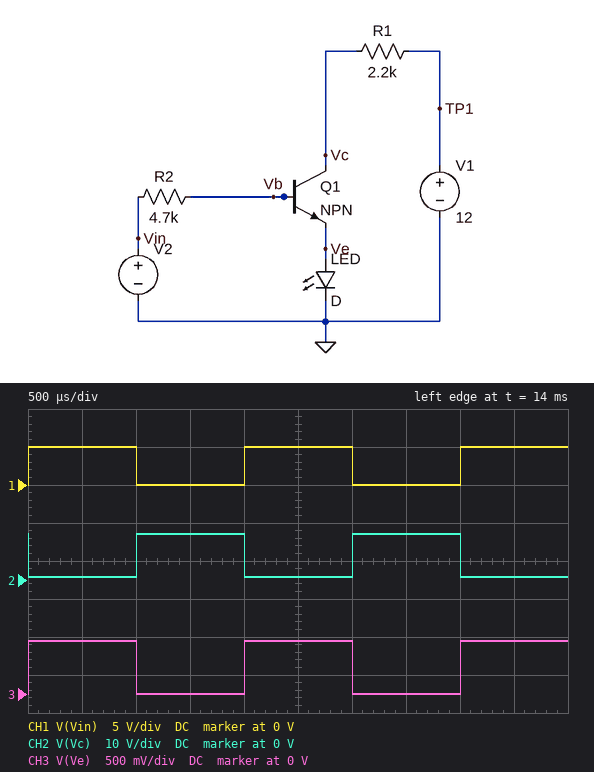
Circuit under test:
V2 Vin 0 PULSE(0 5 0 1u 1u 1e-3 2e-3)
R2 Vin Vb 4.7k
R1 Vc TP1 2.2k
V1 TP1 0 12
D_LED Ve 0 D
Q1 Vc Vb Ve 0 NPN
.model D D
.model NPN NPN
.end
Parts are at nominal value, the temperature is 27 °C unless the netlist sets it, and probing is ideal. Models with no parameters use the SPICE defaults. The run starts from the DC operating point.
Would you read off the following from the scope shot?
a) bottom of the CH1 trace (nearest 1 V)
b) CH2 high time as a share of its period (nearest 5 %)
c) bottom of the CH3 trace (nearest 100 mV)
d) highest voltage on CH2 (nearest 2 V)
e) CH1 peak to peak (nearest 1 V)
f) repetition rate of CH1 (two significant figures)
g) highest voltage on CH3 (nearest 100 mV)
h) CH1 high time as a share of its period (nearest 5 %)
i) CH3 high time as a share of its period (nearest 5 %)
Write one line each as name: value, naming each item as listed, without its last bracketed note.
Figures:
bottom of the CH1 trace: 0 V
CH2 high time as a share of its period: 50 %
bottom of the CH3 trace: 0 V
highest voltage on CH2: 12 V
CH1 peak to peak: 5 V
repetition rate of CH1: 500 Hz
highest voltage on CH3: 700 mV
CH1 high time as a share of its period: 50 %
CH3 high time as a share of its period: 50 %
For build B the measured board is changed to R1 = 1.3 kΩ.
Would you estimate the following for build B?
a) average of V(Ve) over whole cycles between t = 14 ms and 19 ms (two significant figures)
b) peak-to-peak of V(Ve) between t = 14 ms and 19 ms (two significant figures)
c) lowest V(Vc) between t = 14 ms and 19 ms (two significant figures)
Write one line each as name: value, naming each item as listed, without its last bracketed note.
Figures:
average of V(Ve) over whole cycles between t = 14 ms and 19 ms: 360 mV
peak-to-peak of V(Ve) between t = 14 ms and 19 ms: 710 mV
lowest V(Vc) between t = 14 ms and 19 ms: 780 mV
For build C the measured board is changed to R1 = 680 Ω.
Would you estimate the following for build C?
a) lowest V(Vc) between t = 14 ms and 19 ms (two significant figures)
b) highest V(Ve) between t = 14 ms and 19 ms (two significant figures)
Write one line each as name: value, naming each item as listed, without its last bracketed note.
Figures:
lowest V(Vc) between t = 14 ms and 19 ms: 820 mV
highest V(Ve) between t = 14 ms and 19 ms: 730 mV
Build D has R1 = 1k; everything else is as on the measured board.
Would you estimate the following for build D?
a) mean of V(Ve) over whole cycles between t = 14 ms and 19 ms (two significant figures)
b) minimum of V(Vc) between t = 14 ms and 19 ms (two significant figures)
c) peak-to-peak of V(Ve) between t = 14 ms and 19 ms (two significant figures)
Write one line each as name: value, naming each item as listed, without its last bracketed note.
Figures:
mean of V(Ve) over whole cycles between t = 14 ms and 19 ms: 360 mV
minimum of V(Vc) between t = 14 ms and 19 ms: 800 mV
peak-to-peak of V(Ve) between t = 14 ms and 19 ms: 720 mV
